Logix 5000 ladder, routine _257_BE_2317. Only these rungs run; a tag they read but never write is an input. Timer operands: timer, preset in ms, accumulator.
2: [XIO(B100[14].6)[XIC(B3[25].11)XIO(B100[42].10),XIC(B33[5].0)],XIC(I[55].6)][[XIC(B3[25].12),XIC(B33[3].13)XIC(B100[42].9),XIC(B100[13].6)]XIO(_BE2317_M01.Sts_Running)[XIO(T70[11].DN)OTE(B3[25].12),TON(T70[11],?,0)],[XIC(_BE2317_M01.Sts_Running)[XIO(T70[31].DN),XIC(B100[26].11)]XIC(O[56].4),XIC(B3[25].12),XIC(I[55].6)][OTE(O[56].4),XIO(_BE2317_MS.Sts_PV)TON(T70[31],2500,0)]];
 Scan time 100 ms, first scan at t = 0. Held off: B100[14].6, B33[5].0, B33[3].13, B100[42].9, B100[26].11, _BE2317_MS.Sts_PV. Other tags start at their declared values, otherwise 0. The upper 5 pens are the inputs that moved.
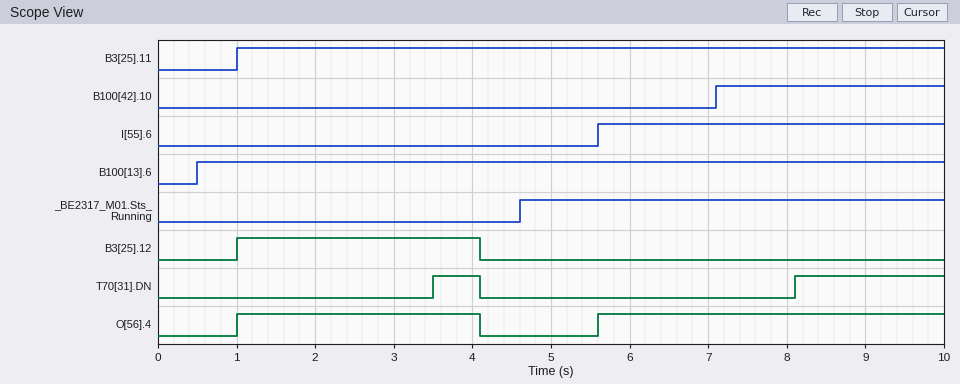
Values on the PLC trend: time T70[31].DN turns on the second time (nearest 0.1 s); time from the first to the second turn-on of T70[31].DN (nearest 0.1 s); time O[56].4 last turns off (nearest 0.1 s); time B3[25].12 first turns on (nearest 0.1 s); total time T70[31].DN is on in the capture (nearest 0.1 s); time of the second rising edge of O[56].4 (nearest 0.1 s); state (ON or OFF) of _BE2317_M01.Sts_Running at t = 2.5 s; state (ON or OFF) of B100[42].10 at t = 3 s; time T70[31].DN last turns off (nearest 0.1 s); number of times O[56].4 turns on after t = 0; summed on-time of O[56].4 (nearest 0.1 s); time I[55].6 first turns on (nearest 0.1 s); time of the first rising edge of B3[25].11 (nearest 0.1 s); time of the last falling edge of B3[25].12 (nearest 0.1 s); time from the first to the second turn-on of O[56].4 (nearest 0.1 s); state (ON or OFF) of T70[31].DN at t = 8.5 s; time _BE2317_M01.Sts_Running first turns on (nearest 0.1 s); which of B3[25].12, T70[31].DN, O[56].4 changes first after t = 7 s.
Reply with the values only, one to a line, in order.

8.1 s
4.6 s
4.1 s
1.0 s
2.5 s
5.6 s
OFF
OFF
4.1 s
2
7.5 s
5.6 s
1.0 s
4.1 s
4.6 s
ON
4.6 s
T70[31].DN
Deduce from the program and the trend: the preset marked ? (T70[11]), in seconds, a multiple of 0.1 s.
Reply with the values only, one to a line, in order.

3.0 s
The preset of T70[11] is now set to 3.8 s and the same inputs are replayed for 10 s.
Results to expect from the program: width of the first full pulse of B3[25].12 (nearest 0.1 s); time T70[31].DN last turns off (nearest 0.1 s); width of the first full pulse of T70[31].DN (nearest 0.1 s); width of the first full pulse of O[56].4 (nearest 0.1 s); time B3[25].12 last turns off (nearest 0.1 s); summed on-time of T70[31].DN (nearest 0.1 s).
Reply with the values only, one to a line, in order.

3.6 s
4.6 s
1.1 s
3.6 s
4.6 s
3.0 s
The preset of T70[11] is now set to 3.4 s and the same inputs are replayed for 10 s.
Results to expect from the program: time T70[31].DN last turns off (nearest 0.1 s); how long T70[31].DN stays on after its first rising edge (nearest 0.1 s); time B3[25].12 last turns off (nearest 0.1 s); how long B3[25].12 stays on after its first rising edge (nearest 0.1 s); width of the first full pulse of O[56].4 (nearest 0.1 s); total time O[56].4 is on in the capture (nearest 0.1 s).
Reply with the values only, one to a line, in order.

4.5 s
1.0 s
4.5 s
3.5 s
3.5 s
7.9 s
